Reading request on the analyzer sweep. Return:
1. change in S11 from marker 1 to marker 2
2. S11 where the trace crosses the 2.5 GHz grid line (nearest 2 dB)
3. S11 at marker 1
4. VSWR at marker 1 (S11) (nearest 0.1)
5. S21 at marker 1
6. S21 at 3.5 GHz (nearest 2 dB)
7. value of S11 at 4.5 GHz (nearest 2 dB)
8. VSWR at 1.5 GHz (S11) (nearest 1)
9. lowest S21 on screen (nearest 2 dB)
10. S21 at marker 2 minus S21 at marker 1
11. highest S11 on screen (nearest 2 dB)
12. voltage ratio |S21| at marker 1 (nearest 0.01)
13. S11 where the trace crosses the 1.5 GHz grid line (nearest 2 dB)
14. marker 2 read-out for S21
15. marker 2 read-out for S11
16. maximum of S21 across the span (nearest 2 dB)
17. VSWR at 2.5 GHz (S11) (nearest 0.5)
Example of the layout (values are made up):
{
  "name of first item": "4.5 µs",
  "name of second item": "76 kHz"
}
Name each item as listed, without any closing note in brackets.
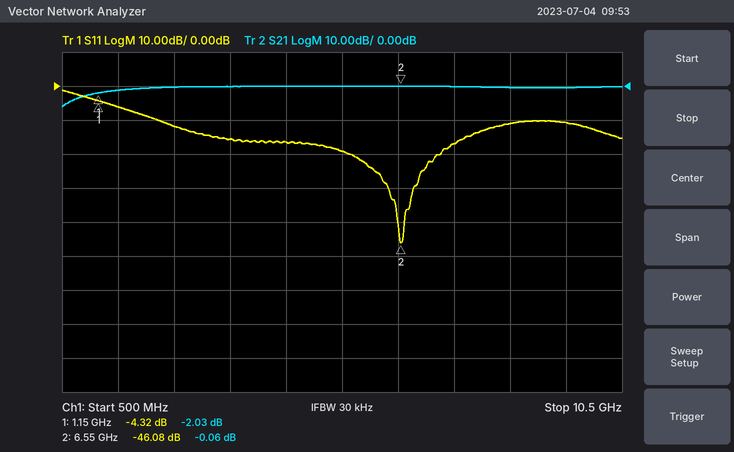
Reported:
{
  "change in S11 from marker 1 to marker 2": "-41.76 dB",
  "S11 where the trace crosses the 2.5 GHz grid line": "-12 dB",
  "S11 at marker 1": "-4.32 dB",
  "VSWR at marker 1 (S11)": "4.1",
  "S21 at marker 1": "-2.03 dB",
  "S21 at 3.5 GHz": "0 dB",
  "value of S11 at 4.5 GHz": "-16 dB",
  "VSWR at 1.5 GHz (S11)": "3",
  "lowest S21 on screen": "-6 dB",
  "S21 at marker 2 minus S21 at marker 1": "1.97 dB",
  "highest S11 on screen": "-2 dB",
  "voltage ratio |S21| at marker 1": "0.79",
  "S11 where the trace crosses the 1.5 GHz grid line": "-6 dB",
  "marker 2 read-out for S21": "-0.06 dB",
  "marker 2 read-out for S11": "-46.08 dB",
  "maximum of S21 across the span": "0 dB",
  "VSWR at 2.5 GHz (S11)": "1.5"
}
